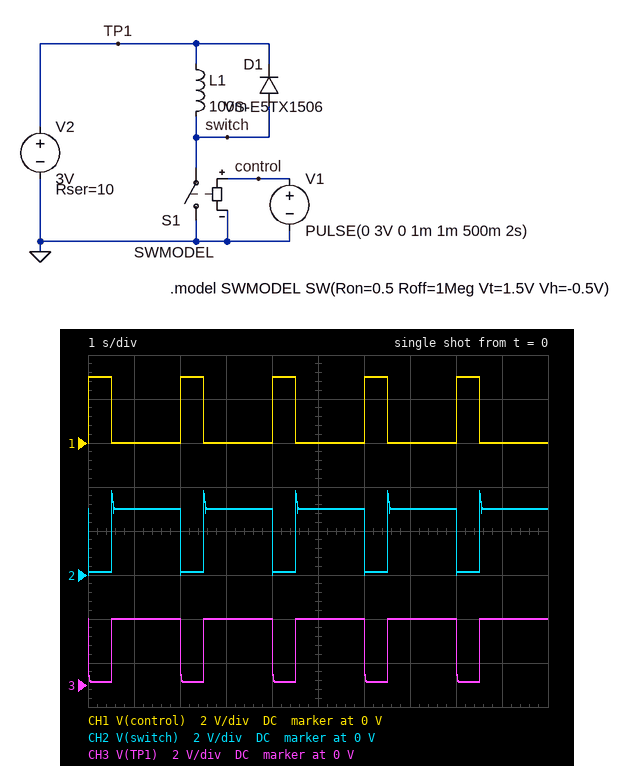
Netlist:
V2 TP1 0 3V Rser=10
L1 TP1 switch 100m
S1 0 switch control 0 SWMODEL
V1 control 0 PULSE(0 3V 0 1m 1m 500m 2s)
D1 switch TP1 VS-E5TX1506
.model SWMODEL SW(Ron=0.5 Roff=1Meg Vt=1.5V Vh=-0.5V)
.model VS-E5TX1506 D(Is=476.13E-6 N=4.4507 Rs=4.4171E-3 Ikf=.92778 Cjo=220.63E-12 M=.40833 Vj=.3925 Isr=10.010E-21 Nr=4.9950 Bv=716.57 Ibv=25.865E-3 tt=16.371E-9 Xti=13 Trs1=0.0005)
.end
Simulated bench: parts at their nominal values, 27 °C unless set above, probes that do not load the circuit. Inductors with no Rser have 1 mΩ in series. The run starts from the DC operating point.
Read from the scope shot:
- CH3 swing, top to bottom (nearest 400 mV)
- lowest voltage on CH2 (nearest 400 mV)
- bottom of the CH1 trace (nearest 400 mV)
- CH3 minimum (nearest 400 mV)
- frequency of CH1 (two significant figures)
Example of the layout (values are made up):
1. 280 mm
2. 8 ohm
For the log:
1. 2.8 V
2. 0 V
3. 0 V
4. 0 V
5. 500 mHz
